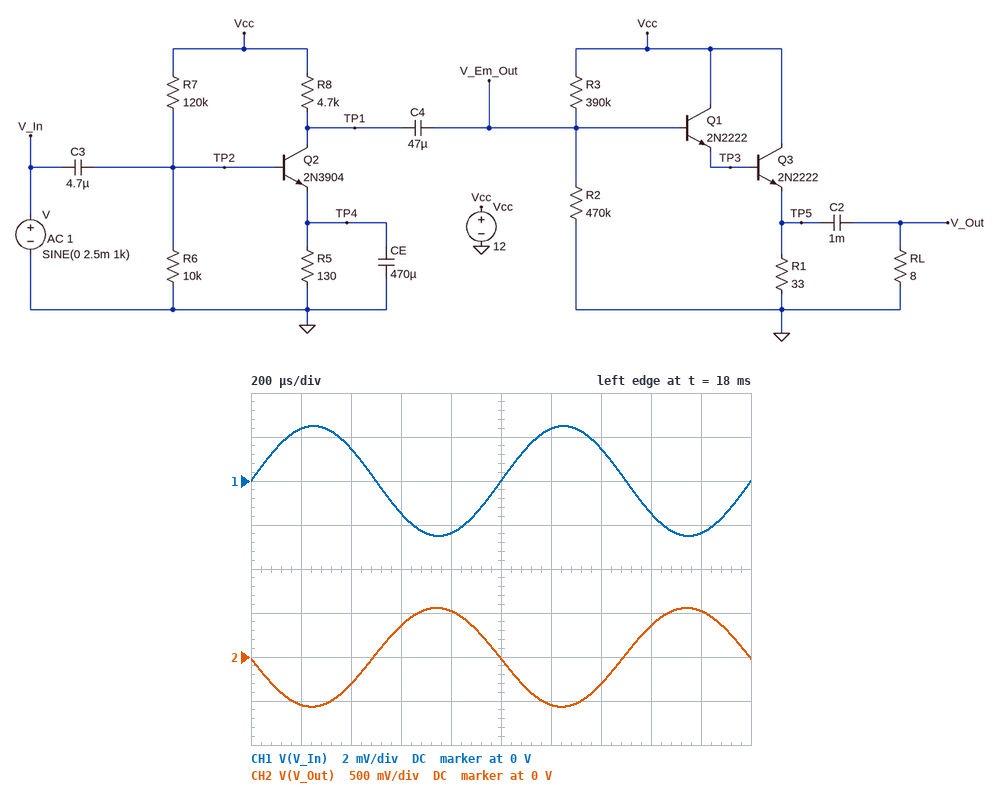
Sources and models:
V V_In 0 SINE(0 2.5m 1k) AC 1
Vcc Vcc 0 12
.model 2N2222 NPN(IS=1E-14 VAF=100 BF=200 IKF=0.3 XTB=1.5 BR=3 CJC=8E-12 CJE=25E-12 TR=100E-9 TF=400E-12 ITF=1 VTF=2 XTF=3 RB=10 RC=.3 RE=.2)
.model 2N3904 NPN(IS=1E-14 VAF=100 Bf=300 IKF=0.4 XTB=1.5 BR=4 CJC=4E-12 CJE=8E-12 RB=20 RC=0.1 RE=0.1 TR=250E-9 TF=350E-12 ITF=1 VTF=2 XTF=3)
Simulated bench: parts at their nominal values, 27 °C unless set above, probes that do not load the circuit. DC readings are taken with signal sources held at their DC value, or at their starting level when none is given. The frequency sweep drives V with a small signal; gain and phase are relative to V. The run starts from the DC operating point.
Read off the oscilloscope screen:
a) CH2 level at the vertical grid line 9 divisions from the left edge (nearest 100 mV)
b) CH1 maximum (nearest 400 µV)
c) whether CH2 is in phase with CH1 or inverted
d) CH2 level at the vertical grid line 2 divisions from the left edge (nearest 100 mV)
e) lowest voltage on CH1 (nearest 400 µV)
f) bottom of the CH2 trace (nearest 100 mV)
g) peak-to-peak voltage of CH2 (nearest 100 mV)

500 mV
2.4 mV
inverted
-300 mV
-2.4 mV
-600 mV
1.1 V
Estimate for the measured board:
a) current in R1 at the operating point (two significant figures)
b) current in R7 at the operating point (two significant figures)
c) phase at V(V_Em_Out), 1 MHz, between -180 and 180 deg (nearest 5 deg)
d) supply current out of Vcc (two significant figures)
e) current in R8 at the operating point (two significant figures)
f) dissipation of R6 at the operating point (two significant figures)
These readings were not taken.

130 mA
93 µA
165 deg
130 mA
1.6 mA
77 µW
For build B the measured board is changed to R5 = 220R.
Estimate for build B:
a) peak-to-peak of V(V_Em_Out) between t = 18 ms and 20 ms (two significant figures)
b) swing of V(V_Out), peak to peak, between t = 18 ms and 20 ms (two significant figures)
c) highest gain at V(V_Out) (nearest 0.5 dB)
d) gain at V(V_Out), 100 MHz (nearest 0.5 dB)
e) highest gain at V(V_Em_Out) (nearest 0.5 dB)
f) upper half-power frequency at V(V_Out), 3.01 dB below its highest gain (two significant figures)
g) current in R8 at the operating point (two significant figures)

880 mV
780 mV
44.0 dB
0 dB
45.0 dB
4.6 MHz
1.1 mA
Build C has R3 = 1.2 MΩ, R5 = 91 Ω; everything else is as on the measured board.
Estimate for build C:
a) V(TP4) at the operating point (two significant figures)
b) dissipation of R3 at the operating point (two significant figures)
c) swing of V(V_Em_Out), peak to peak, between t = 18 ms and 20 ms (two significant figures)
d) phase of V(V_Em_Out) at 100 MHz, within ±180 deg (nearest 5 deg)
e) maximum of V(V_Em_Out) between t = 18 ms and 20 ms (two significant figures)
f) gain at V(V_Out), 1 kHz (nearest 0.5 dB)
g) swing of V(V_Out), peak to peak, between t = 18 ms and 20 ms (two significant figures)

190 mV
68 µW
1.6 V
75 deg
3.8 V
48.5 dB
920 mV
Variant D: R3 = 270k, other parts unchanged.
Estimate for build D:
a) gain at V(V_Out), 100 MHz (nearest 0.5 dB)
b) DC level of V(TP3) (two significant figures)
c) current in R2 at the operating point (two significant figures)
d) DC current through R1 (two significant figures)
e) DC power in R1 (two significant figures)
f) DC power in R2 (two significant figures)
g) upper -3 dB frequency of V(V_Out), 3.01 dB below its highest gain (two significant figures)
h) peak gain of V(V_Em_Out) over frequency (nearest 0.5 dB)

3.5 dB
6.1 V
14 µA
160 mA
830 mW
96 µW
3.9 MHz
48.0 dB
